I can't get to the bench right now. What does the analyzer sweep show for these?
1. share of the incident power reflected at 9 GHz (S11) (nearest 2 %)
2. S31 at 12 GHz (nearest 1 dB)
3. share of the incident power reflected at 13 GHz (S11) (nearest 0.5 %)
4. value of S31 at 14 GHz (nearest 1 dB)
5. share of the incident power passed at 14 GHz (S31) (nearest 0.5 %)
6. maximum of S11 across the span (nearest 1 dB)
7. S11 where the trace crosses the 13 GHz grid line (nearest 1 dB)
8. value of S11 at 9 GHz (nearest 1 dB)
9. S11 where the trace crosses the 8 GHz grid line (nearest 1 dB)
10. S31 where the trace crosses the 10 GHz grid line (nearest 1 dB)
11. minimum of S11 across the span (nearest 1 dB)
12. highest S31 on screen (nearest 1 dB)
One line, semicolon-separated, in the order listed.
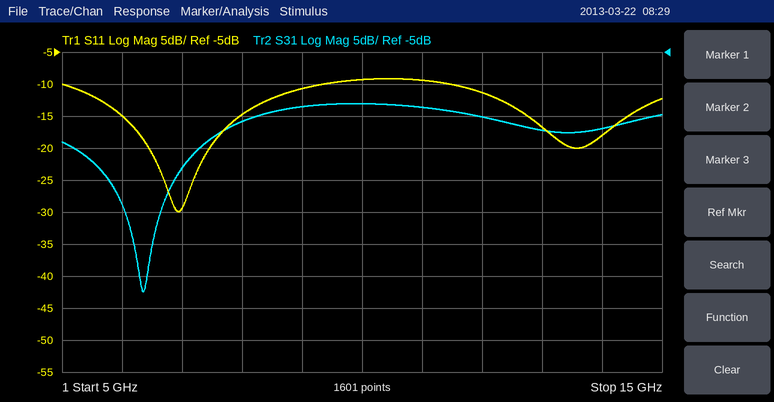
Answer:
8 %; -15 dB; 2.0 %; -17 dB; 2.0 %; -9 dB; -17 dB; -11 dB; -15 dB; -13 dB; -30 dB; -13 dB
